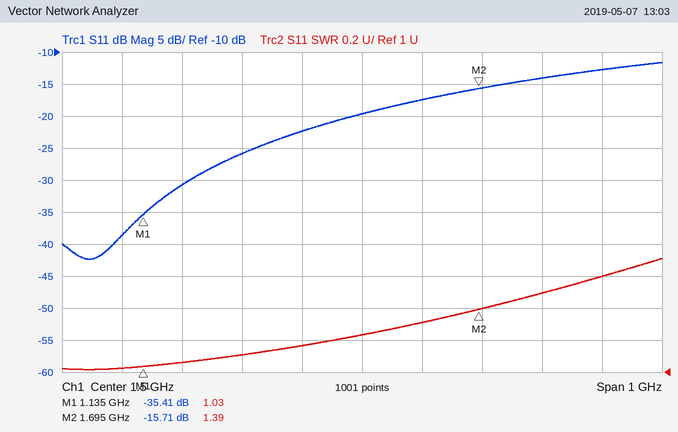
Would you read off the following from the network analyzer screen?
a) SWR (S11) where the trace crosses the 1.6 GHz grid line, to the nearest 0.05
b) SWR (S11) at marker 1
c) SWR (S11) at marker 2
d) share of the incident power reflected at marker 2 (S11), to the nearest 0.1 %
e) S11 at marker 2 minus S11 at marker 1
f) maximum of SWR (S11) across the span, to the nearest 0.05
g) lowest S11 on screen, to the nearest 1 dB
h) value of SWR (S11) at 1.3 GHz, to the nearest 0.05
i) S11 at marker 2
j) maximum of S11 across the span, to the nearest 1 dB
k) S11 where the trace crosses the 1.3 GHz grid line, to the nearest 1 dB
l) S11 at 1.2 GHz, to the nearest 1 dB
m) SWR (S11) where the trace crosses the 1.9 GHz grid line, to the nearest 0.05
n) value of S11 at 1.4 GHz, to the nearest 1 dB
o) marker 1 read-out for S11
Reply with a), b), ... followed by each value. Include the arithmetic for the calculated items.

a) 1.30
b) 1.03
c) 1.39
d) 10^(-15.71/10) ≈ 2.7 %
e) -15.71 − (-35.41) = 19.70 dB
f) 1.70
g) -42 dB
h) 1.10
i) -15.71 dB
j) -12 dB
k) -26 dB
l) -31 dB
m) 1.60
n) -22 dB
o) -35.41 dB
